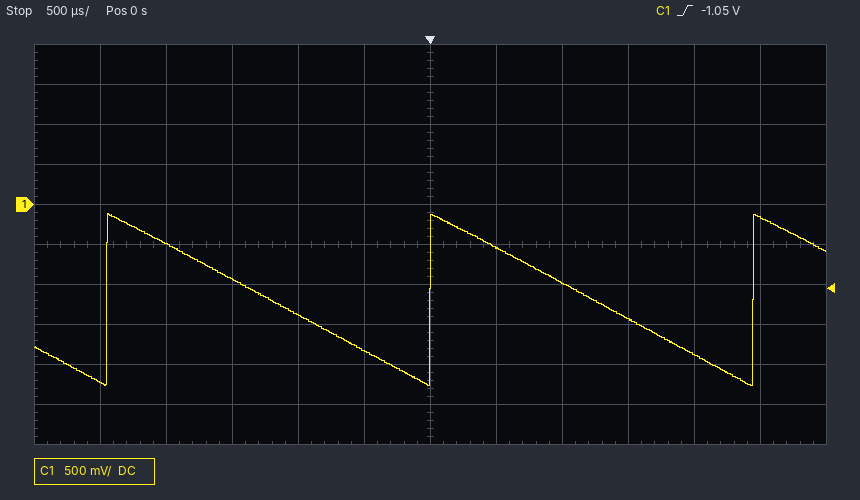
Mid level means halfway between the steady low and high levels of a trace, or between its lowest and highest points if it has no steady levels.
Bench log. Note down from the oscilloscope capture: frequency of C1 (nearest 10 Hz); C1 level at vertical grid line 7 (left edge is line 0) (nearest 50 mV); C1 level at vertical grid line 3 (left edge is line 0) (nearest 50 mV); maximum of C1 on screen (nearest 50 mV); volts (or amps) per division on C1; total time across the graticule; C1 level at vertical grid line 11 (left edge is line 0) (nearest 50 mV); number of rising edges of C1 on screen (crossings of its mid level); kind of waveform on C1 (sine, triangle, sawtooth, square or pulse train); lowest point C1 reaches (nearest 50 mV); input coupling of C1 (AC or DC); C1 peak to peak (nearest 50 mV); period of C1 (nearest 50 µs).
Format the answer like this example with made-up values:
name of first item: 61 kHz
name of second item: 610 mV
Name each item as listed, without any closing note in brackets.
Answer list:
frequency of C1: 410 Hz
C1 level at vertical grid line 7 (left edge is line 0): -550 mV
C1 level at vertical grid line 3 (left edge is line 0): -950 mV
maximum of C1 on screen: -100 mV
volts (or amps) per division on C1: 500 mV
total time across the graticule: 6 ms
C1 level at vertical grid line 11 (left edge is line 0): -150 mV
number of rising edges of C1 on screen: 3
kind of waveform on C1: sawtooth
lowest point C1 reaches: -2.25 V
input coupling of C1: DC
C1 peak to peak: 2.15 V
period of C1: 2.45 ms
